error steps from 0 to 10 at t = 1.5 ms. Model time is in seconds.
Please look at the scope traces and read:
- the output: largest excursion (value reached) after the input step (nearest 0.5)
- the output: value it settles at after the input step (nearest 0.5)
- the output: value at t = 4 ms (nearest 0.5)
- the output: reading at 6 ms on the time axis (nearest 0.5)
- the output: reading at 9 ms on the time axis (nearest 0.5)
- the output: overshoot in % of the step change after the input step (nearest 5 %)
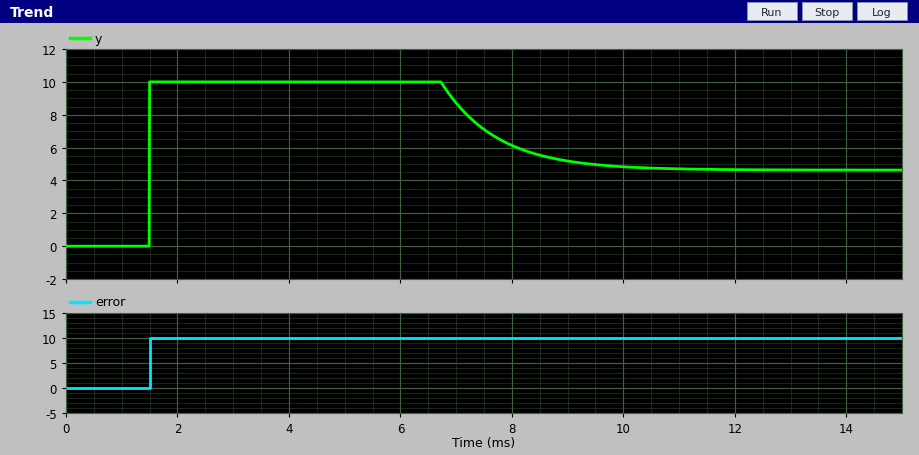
10.0
4.5
10.0
10.0
5.0
115 %
